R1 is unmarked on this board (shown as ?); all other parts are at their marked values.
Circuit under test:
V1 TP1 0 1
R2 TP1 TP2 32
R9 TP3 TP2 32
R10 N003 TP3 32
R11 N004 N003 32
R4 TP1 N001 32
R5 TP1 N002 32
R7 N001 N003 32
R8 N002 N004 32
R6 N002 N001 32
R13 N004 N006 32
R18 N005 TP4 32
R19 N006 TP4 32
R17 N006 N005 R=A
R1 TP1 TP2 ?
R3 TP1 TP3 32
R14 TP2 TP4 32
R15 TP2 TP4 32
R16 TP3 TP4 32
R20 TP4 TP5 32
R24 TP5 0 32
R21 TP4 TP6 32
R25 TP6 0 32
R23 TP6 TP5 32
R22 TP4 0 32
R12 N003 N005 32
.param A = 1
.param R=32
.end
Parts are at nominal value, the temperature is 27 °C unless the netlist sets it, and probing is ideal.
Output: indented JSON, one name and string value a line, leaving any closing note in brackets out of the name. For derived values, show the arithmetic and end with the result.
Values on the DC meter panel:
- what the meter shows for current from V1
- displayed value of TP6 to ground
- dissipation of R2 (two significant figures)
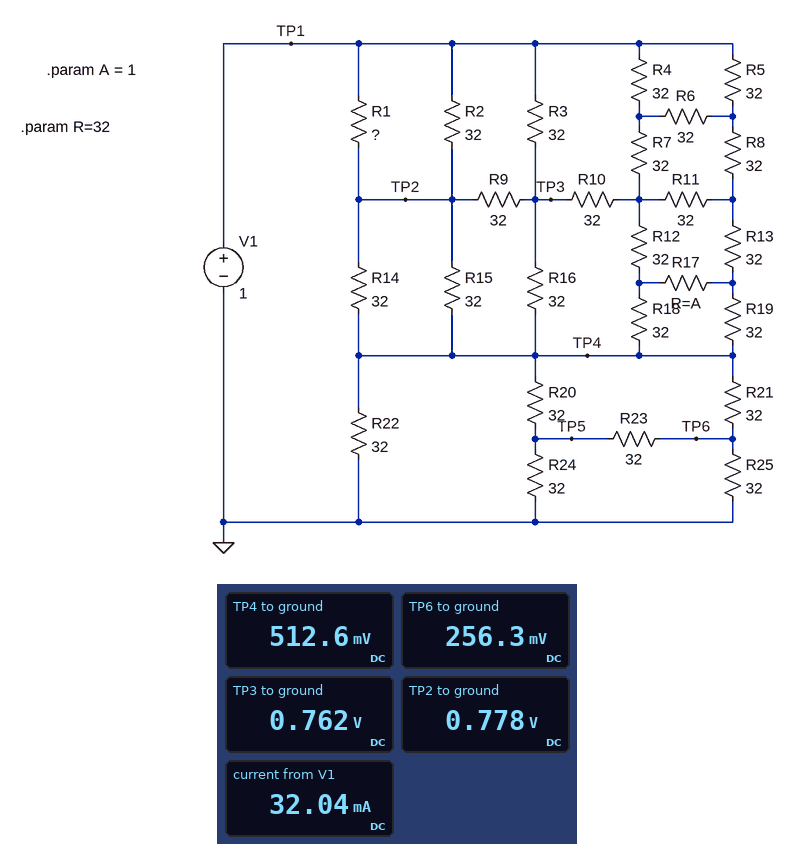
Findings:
{
  "what the meter shows for current from V1": "32.04 mA",
  "displayed value of TP6 to ground": "256.3 mV",
  "dissipation of R2": "(1 V - 778 mV)^2 / 32 Ω = 1.5 mW"
}
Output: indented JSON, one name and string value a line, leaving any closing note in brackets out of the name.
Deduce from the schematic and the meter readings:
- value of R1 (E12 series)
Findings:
{
  "value of R1": "22 Ω"
}
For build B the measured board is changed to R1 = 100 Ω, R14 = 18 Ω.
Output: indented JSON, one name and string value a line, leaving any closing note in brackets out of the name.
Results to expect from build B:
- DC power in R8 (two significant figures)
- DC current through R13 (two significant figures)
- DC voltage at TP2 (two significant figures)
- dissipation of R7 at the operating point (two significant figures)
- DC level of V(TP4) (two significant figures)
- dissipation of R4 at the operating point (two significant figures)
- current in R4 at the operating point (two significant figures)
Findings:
{
  "DC power in R8": "530 µW",
  "DC current through R13": "3.9 mA",
  "DC voltage at TP2": "670 mV",
  "dissipation of R7 at the operating point": "550 µW",
  "DC level of V(TP4)": "490 mV",
  "dissipation of R4 at the operating point": "540 µW",
  "current in R4 at the operating point": "4.1 mA"
}
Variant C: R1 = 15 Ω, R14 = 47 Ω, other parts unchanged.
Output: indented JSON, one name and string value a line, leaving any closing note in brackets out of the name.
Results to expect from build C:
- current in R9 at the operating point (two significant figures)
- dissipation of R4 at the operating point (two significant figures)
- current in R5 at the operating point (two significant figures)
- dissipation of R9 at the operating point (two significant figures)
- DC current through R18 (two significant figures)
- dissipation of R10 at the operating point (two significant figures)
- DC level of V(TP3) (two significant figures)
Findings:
{
  "current in R9 at the operating point": "1.4 mA",
  "dissipation of R4 at the operating point": "440 µW",
  "current in R5 at the operating point": "3.7 mA",
  "dissipation of R9 at the operating point": "67 µW",
  "DC current through R18": "3.9 mA",
  "dissipation of R10 at the operating point": "3.7 µW",
  "DC level of V(TP3)": "770 mV"
}
